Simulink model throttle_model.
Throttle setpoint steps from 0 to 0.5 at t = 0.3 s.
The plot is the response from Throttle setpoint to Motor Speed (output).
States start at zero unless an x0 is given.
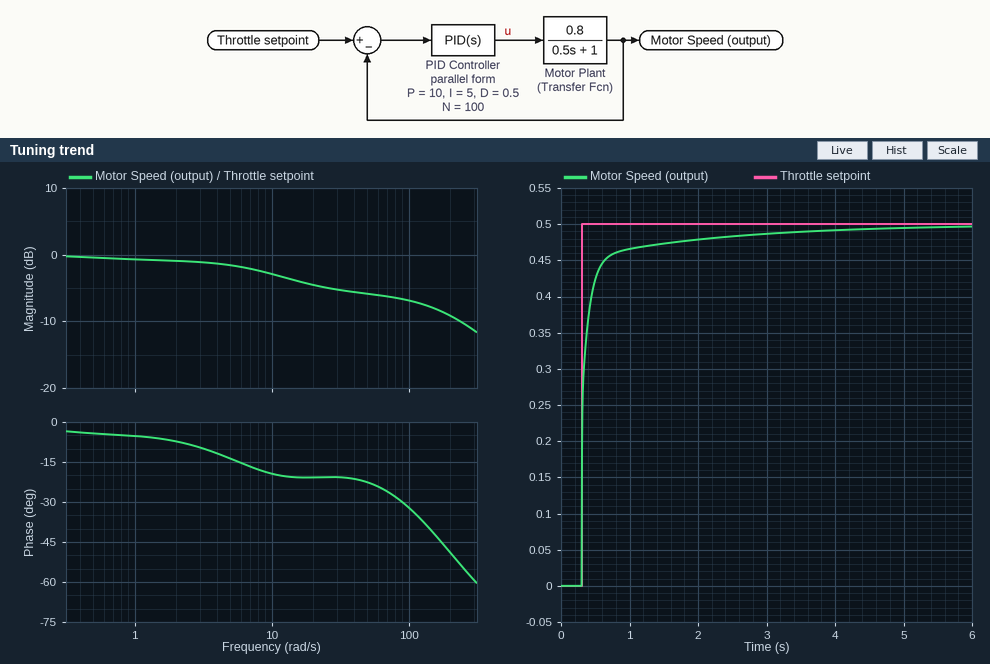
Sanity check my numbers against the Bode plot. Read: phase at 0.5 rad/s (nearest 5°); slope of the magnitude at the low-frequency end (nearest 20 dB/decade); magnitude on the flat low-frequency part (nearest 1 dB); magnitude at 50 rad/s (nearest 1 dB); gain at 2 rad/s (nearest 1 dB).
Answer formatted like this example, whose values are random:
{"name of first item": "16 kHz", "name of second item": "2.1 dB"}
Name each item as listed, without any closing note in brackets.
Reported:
{"phase at 0.5 rad/s": "-5°", "slope of the magnitude at the low-frequency end": "0 dB/decade", "magnitude on the flat low-frequency part": "0 dB", "magnitude at 50 rad/s": "-6 dB", "gain at 2 rad/s": "-1 dB"}
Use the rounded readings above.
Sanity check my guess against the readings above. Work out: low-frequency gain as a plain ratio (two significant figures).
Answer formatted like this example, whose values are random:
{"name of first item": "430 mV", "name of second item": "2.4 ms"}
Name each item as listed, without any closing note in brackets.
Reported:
{"low-frequency gain as a plain ratio": "1.0"}
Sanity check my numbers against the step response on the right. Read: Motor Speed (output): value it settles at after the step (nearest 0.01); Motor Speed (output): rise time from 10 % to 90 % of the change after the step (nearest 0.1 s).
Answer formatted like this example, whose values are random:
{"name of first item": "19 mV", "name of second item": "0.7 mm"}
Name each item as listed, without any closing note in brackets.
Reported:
{"Motor Speed (output): value it settles at after the step": "0.50", "Motor Speed (output): rise time from 10 % to 90 % of the change after the step": "0.3 s"}
